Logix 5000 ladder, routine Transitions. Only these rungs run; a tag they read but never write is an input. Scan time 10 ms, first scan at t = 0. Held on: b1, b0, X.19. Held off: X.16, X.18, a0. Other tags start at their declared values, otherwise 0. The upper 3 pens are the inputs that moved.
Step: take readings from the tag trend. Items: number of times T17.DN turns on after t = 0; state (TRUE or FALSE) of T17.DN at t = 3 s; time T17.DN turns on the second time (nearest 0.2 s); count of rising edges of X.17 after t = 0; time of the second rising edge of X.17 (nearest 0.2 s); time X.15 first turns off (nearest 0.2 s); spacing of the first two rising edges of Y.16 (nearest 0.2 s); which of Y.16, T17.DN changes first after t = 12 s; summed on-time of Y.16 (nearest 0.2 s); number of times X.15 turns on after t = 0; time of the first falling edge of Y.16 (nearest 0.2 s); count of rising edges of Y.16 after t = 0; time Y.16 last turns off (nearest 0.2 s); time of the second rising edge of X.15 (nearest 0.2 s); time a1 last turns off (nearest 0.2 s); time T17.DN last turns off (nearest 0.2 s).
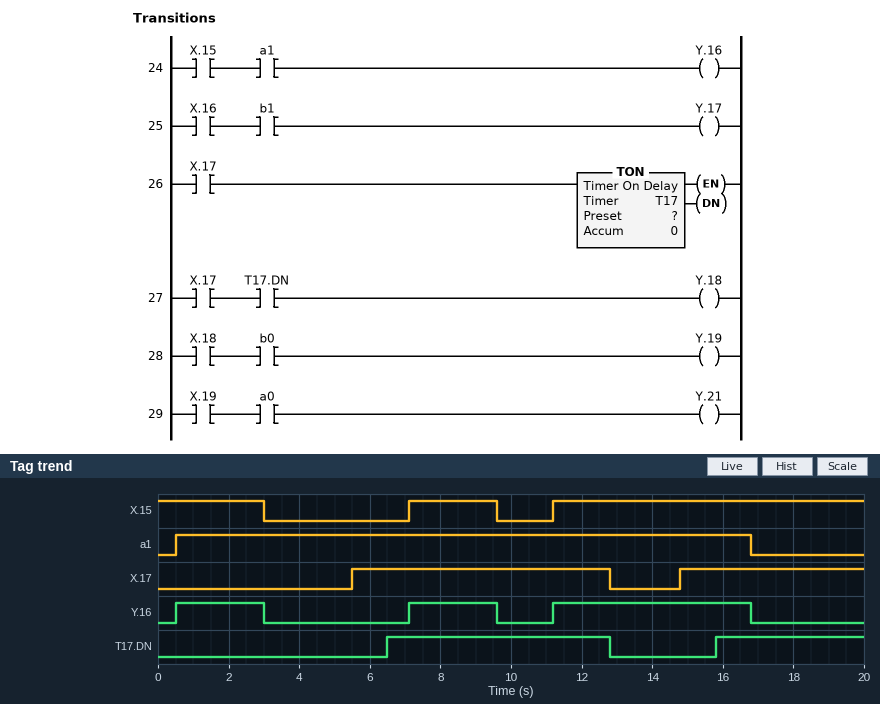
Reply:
2
FALSE
15.8 s
2
14.8 s
3.0 s
6.6 s
T17.DN
10.6 s
2
3.0 s
3
16.8 s
11.2 s
16.8 s
12.8 s
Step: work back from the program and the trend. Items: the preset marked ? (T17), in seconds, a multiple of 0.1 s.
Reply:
1.0 s
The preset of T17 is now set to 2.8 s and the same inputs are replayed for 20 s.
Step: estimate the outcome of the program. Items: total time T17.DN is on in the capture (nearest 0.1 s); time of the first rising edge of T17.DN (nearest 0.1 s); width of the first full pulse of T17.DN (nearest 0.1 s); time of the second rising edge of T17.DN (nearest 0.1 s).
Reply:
6.9 s
8.3 s
4.5 s
17.6 s
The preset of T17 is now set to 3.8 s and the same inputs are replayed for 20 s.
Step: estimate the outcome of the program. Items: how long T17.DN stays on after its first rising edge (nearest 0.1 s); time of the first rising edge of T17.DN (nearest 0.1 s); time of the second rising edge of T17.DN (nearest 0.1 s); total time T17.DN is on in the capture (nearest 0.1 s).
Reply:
3.5 s
9.3 s
18.6 s
4.9 s
